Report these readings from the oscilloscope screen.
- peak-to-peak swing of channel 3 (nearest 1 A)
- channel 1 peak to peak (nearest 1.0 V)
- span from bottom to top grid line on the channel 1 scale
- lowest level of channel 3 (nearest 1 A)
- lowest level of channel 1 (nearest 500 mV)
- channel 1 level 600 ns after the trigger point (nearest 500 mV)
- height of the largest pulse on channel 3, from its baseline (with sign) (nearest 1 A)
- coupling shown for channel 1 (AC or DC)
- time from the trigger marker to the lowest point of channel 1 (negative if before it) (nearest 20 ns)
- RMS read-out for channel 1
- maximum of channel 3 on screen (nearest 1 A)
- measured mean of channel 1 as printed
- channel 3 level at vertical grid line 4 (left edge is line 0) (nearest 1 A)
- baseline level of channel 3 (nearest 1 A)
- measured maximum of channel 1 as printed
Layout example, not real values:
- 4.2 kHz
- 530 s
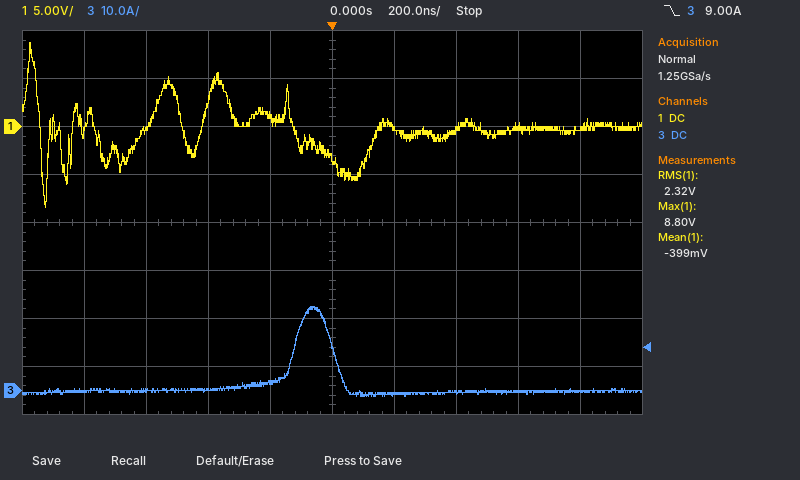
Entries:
- 19 A
- 17.0 V
- 40 V
- -1 A
- -8.5 V
- 0.0 V
- +18 A
- DC
- -920 ns
- 2.32 V
- 18 A
- -399 mV
- 2 A
- 0 A
- 8.80 V
